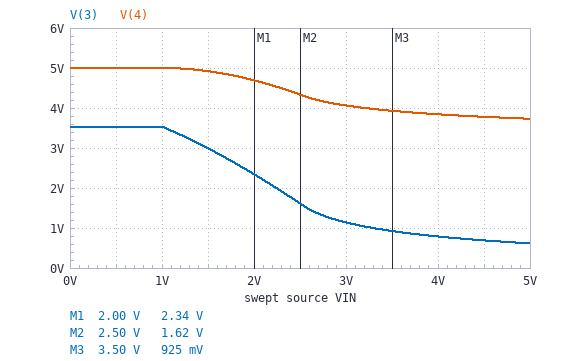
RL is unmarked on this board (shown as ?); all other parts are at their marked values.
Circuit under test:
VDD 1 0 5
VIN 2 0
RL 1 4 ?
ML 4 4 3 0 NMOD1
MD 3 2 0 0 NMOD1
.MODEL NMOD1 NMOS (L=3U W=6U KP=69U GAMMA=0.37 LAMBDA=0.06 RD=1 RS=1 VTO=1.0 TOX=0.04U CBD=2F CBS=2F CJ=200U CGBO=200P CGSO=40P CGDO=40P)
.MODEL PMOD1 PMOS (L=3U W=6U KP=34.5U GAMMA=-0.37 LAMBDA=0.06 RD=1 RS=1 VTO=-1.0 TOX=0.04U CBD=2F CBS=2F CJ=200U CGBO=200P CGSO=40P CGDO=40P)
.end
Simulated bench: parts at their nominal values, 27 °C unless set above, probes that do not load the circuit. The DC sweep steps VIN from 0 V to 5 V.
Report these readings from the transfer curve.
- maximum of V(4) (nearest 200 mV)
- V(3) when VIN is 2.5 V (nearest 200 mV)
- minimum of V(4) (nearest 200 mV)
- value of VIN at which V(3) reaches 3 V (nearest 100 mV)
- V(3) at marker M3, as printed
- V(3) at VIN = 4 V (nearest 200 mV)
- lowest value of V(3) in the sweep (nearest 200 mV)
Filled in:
5.0 V
1.6 V
3.8 V
1.5 V
925 mV
800 mV
600 mV
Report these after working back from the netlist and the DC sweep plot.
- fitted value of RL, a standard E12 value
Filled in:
3.9 kΩ
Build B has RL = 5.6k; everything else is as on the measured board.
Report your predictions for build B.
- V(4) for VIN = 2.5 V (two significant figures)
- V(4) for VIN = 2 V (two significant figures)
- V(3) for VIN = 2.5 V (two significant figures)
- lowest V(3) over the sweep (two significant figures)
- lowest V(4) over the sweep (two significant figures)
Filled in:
4.1 V
4.6 V
1.4 V
520 mV
3.5 V
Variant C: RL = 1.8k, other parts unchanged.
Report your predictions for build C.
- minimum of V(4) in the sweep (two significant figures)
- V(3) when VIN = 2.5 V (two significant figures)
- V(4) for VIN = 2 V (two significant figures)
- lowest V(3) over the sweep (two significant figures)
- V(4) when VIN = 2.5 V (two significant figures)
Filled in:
4.2 V
1.9 V
4.9 V
820 mV
4.7 V
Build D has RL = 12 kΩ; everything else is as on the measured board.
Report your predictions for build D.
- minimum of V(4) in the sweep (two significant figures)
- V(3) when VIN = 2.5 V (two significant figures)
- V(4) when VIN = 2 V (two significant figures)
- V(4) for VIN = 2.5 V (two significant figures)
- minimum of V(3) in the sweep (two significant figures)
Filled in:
2.9 V
890 mV
4.1 V
3.4 V
330 mV
